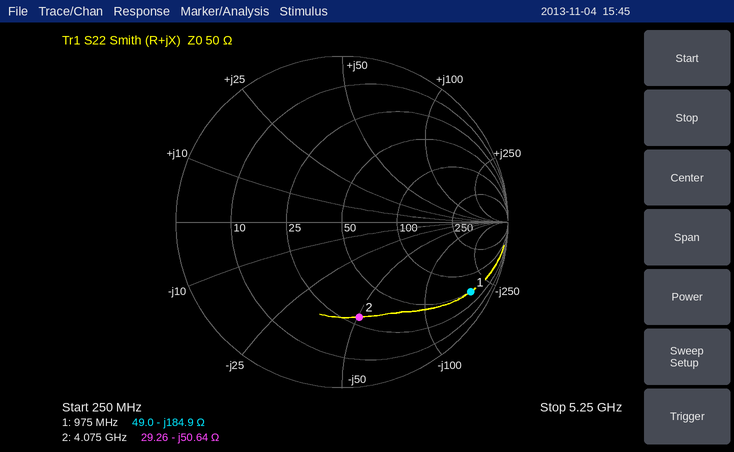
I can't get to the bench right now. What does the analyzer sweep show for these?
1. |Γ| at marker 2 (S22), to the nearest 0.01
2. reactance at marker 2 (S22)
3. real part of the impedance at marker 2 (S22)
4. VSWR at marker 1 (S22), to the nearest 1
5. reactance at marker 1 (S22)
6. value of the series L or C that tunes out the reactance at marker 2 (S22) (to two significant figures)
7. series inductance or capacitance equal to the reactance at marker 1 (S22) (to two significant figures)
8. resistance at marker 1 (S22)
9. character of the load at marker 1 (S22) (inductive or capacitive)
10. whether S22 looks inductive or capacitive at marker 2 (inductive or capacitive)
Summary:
0.58
-50.64 Ω
29.26 Ω
16
-184.9 Ω
2.0 nH
880 fF
49.0 Ω
capacitive
capacitive
